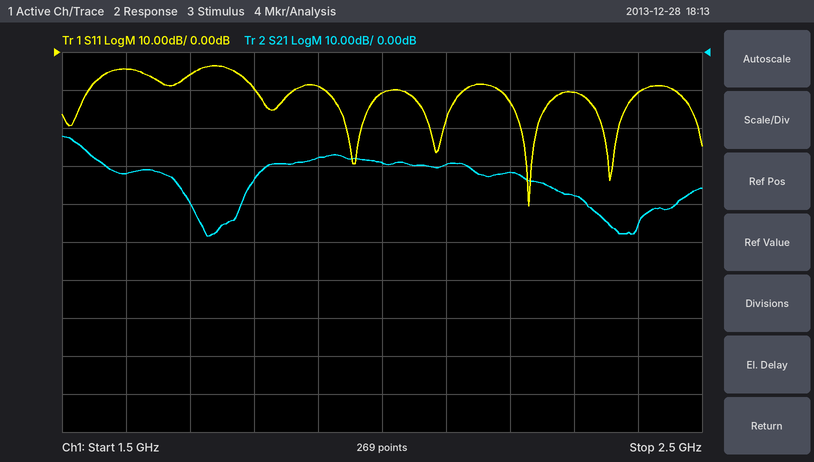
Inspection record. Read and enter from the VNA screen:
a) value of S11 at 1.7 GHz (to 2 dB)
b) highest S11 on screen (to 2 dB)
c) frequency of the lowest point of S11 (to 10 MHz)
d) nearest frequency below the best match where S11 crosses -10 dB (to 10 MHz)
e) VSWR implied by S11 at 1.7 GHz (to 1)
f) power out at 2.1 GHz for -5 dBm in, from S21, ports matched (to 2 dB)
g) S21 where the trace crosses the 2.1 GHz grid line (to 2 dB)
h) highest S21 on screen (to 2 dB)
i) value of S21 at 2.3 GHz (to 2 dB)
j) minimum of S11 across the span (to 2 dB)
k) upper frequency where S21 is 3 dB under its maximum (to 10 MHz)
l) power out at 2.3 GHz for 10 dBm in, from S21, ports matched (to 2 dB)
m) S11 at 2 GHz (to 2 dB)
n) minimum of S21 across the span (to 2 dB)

-6 dB
-4 dB
2.23 GHz
2.18 GHz
3
-34 dBm
-30 dB
-22 dB
-38 dB
-40 dB
1.53 GHz
-28 dBm
-10 dB
-48 dB
